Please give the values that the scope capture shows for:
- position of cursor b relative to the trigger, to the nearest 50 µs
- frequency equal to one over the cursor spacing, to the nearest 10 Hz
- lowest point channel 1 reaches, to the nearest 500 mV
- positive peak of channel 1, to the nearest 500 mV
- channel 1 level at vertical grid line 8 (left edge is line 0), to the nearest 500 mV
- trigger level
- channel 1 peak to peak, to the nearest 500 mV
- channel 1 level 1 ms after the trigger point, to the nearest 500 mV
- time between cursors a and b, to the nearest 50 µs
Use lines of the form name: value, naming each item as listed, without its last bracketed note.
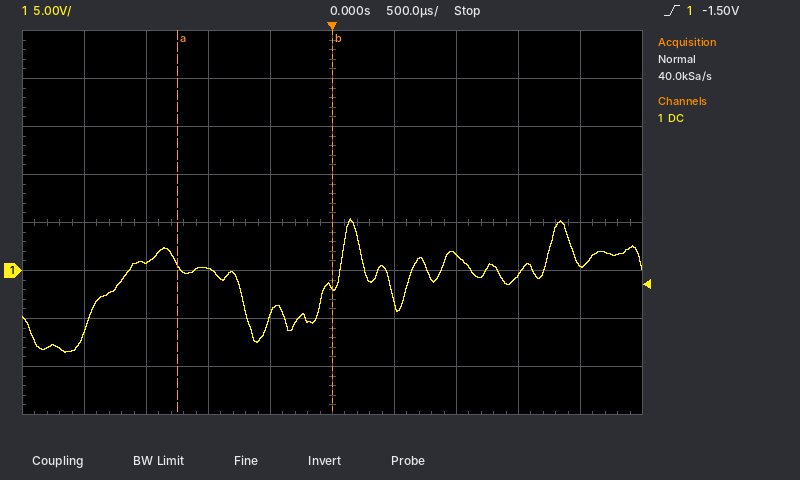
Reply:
position of cursor b relative to the trigger, to the nearest 50 µs: 0 µs
frequency equal to one over the cursor spacing, to the nearest 10 Hz: 800 Hz
lowest point channel 1 reaches, to the nearest 500 mV: -8.5 V
positive peak of channel 1, to the nearest 500 mV: 5.5 V
channel 1 level at vertical grid line 8 (left edge is line 0), to the nearest 500 mV: -500 mV
trigger level: -1.50 V
channel 1 peak to peak, to the nearest 500 mV: 14.0 V
channel 1 level 1 ms after the trigger point, to the nearest 500 mV: 1.5 V
time between cursors a and b, to the nearest 50 µs: 1.25 ms
